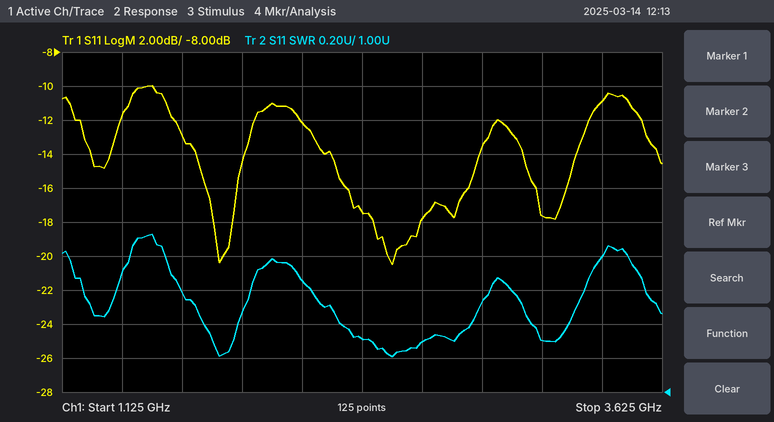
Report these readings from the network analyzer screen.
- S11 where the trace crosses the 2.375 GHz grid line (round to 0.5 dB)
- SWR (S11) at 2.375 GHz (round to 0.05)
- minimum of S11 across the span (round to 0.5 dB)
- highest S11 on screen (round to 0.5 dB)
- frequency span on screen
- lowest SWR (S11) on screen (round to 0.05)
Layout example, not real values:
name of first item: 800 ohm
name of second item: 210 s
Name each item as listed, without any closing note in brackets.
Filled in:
S11 where the trace crosses the 2.375 GHz grid line: -17.5 dB
SWR (S11) at 2.375 GHz: 1.30
minimum of S11 across the span: -20.5 dB
highest S11 on screen: -10.0 dB
frequency span on screen: 2.5 GHz
lowest SWR (S11) on screen: 1.20
